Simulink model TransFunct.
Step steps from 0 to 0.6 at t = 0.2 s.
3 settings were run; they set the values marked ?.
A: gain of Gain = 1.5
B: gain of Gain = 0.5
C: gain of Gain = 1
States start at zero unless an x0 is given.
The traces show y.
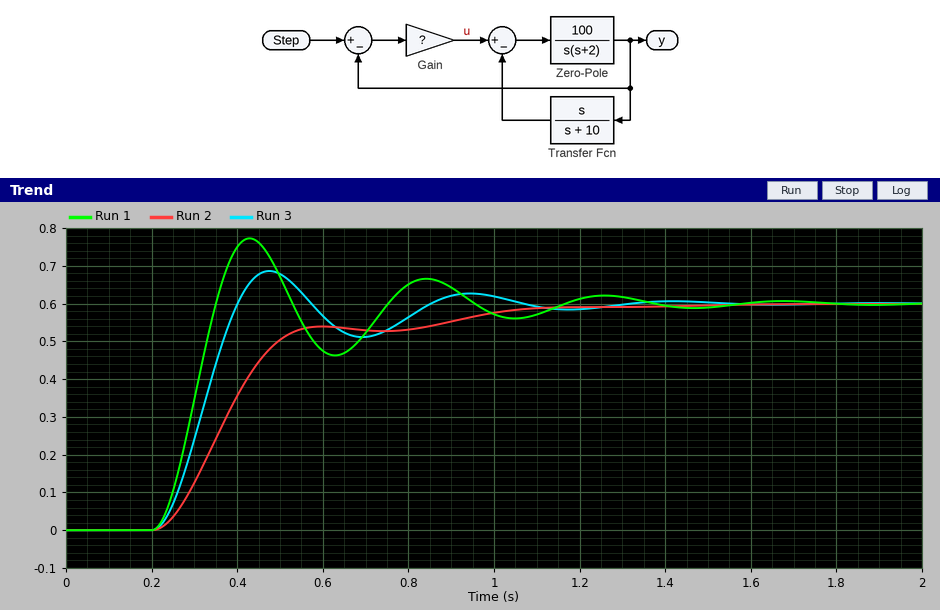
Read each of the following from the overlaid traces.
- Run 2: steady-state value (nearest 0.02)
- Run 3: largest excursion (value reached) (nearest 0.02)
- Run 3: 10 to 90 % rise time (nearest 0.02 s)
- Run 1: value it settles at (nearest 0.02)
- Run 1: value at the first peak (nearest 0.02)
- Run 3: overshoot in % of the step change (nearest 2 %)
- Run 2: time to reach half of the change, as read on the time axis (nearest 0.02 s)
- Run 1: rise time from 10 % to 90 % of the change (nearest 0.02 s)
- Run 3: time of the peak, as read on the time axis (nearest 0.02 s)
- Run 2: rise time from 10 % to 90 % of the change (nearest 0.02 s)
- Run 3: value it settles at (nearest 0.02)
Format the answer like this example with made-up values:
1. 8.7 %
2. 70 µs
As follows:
1. 0.60
2. 0.68
3. 0.14 s
4. 0.60
5. 0.78
6. 14 %
7. 0.38 s
8. 0.10 s
9. 0.48 s
10. 0.58 s
11. 0.60
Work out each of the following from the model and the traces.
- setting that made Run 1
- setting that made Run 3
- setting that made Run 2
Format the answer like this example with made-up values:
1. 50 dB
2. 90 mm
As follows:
1. A
2. C
3. B
